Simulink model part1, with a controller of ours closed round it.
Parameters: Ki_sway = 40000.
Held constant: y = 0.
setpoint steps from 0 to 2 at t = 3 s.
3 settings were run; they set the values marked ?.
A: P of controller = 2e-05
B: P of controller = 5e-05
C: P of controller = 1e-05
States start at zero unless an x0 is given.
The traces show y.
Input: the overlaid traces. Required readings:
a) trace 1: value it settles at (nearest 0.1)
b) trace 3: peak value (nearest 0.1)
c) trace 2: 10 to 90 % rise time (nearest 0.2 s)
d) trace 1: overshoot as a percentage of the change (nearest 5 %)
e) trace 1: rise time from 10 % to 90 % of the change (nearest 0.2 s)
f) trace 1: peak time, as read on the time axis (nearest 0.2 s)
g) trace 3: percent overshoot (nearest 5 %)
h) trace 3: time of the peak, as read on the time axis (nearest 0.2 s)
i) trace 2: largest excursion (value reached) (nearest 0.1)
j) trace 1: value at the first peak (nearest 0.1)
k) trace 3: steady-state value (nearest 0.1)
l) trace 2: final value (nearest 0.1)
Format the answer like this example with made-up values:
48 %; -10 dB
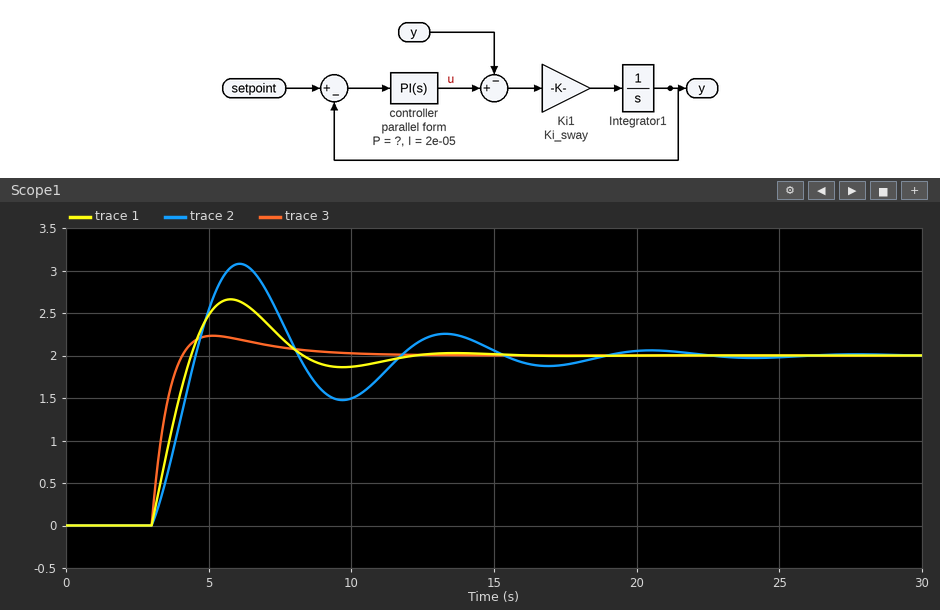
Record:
2.0; 2.2; 1.2 s; 35 %; 1.0 s; 5.8 s; 10 %; 5.2 s; 3.1; 2.7; 2.0; 2.0
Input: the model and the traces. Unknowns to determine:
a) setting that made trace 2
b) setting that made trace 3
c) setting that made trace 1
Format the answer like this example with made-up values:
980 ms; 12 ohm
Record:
C; B; A
